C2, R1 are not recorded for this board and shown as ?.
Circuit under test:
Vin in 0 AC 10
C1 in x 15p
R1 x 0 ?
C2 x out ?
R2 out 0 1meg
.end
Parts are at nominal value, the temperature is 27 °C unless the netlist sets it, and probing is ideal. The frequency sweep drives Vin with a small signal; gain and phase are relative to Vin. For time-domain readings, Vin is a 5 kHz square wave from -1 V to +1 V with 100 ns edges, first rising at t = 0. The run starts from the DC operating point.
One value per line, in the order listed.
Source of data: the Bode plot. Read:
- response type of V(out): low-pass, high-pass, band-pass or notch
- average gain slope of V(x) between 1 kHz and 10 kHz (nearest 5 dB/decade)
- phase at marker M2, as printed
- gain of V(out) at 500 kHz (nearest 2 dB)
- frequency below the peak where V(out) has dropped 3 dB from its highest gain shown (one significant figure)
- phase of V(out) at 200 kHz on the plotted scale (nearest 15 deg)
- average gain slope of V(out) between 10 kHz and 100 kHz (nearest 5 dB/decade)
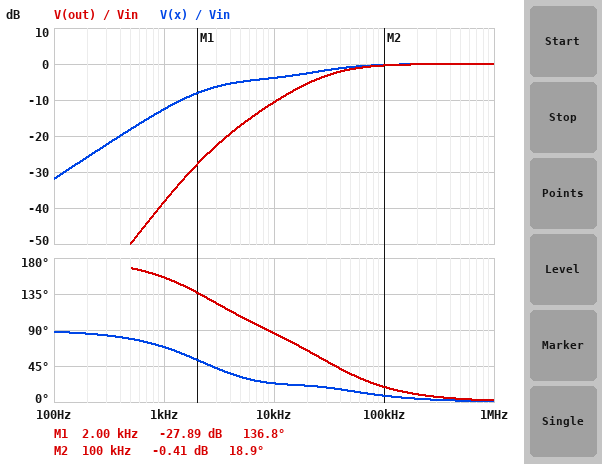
high-pass
10 dB/decade
18.9 deg
0 dB
30 kHz
15 deg
10 dB/decade
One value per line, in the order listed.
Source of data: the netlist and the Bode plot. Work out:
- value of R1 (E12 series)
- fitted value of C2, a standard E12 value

2.7 MΩ
8.2 pF
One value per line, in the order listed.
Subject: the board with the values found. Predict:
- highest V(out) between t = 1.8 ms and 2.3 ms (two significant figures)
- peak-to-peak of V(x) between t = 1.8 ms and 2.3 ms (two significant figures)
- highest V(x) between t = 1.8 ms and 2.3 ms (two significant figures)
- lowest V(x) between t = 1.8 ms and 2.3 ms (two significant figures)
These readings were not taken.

2.0 V
3.6 V
1.8 V
-1.8 V
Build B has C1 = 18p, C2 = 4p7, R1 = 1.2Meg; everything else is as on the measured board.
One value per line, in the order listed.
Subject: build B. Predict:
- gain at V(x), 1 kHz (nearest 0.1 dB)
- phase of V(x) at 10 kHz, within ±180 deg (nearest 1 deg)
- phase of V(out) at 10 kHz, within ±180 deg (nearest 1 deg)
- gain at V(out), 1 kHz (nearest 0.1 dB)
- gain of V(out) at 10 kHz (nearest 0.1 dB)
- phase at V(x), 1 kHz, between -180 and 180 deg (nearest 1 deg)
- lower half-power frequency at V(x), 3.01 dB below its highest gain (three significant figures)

-17.5 dB
33 deg
107 deg
-48.1 dB
-14.4 dB
80 deg
12.0 kHz
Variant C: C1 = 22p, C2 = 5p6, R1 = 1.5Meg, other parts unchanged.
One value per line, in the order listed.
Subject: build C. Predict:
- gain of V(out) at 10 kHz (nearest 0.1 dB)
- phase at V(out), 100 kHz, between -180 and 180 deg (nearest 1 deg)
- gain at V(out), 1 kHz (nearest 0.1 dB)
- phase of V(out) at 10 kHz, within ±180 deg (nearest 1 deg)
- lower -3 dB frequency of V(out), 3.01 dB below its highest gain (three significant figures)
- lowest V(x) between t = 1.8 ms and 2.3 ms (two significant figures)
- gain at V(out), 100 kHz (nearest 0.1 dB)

-12.2 dB
22 deg
-43.0 dB
95 deg
37.1 kHz
-1.9 V
-0.6 dB
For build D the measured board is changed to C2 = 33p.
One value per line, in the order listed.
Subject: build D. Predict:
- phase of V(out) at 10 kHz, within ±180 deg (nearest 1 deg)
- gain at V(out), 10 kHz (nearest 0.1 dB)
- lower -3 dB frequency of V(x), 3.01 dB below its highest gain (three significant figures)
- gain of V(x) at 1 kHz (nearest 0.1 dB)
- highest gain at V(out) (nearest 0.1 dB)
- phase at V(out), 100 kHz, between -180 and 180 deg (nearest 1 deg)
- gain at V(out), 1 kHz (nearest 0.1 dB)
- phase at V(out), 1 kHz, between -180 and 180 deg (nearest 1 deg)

67 deg
-6.4 dB
17.1 kHz
-14.6 dB
0 dB
11 deg
-28.4 dB
133 deg
